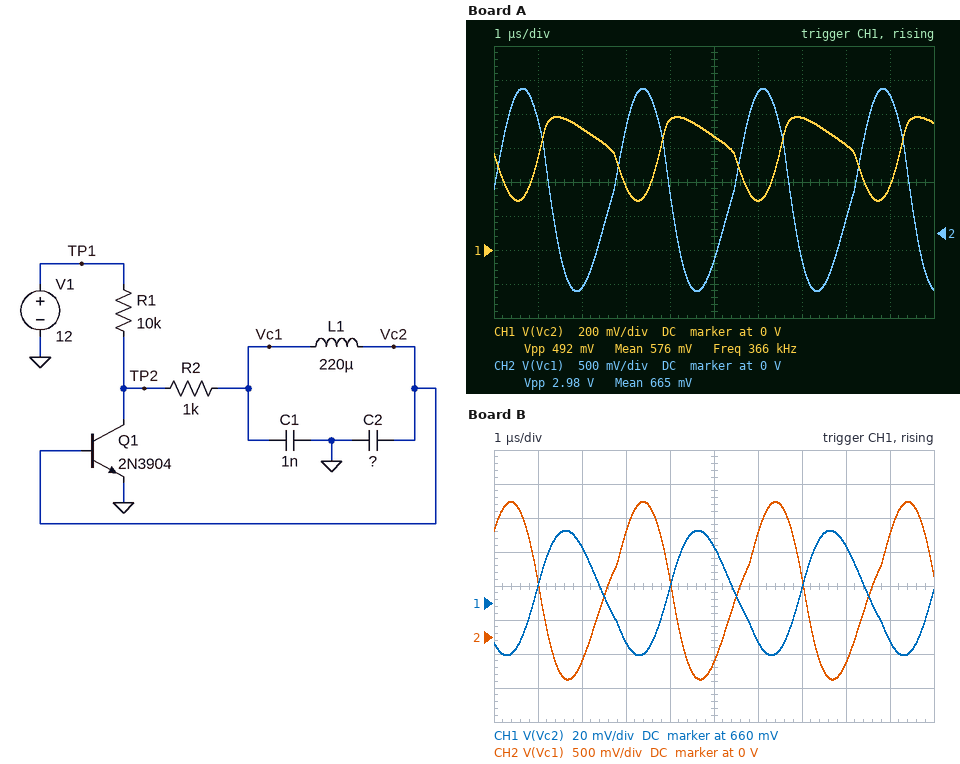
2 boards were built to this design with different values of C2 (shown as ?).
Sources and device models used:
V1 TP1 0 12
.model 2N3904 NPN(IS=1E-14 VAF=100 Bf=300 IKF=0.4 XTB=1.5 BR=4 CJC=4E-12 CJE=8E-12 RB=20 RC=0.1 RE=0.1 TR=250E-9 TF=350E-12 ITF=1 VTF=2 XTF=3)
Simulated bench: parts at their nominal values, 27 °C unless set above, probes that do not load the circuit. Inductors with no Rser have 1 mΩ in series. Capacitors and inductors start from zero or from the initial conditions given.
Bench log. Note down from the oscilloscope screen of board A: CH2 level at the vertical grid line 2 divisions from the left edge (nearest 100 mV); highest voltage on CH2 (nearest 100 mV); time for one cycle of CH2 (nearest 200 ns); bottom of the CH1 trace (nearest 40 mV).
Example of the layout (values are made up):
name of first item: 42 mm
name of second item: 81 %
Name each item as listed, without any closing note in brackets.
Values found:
CH2 level at the vertical grid line 2 divisions from the left edge: -800 mV
highest voltage on CH2: 2.1 V
time for one cycle of CH2: 2.8 µs
bottom of the CH1 trace: 280 mV
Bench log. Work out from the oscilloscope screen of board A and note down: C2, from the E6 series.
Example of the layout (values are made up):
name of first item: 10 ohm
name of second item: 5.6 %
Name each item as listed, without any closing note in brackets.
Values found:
C2, from the E6 series: 3.3 nF
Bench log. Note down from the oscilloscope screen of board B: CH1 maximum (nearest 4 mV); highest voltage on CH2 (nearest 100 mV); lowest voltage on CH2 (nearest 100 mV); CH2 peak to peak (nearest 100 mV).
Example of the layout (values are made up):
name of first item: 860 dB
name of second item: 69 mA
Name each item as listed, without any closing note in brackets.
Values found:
CH1 maximum: 704 mV
highest voltage on CH2: 2.0 V
lowest voltage on CH2: -600 mV
CH2 peak to peak: 2.6 V
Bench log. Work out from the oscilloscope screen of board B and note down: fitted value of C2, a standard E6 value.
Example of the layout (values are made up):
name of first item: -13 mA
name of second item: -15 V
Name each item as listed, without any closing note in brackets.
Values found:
fitted value of C2, a standard E6 value: 33 nF
